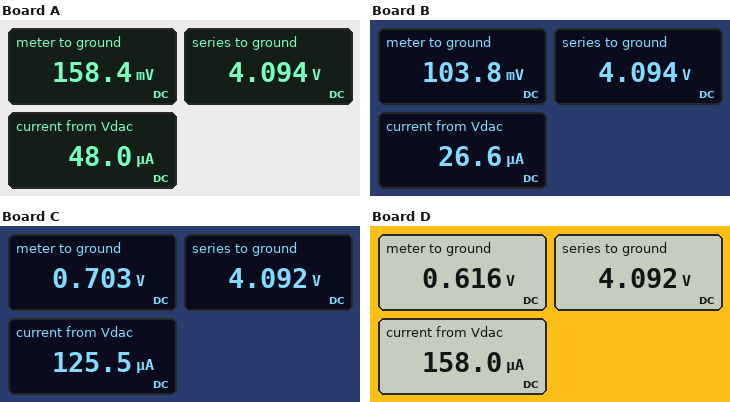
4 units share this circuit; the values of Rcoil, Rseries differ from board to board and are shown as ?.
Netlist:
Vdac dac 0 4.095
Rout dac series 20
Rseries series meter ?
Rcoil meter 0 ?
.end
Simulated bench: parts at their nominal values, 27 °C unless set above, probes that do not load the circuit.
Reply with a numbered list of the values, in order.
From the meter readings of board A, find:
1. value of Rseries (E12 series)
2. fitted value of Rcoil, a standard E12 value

1. 82 kΩ
2. 3.3 kΩ
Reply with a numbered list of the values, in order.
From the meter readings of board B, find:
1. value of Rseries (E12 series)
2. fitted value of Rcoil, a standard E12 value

1. 150 kΩ
2. 3.9 kΩ
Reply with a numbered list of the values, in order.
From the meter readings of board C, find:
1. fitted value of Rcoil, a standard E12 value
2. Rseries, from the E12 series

1. 5.6 kΩ
2. 27 kΩ
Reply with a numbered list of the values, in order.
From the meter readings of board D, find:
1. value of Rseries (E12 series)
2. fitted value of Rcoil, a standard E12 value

1. 22 kΩ
2. 3.9 kΩ
